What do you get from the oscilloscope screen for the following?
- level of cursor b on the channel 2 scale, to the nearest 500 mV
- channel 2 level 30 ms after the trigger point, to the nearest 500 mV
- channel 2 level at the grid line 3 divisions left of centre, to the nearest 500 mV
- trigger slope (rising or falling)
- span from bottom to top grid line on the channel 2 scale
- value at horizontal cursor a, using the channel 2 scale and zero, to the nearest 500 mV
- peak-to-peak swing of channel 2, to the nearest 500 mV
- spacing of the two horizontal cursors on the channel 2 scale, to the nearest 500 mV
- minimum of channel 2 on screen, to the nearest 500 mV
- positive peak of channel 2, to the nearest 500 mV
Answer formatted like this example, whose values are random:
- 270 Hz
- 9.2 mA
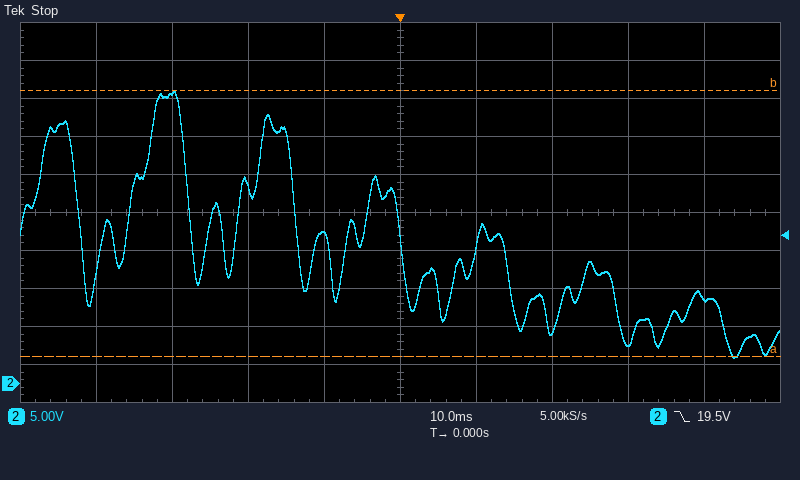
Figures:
- 38.5 V
- 5.5 V
- 38.0 V
- falling
- 50 V
- 3.5 V
- 35.0 V
- 35.0 V
- 3.5 V
- 38.5 V
